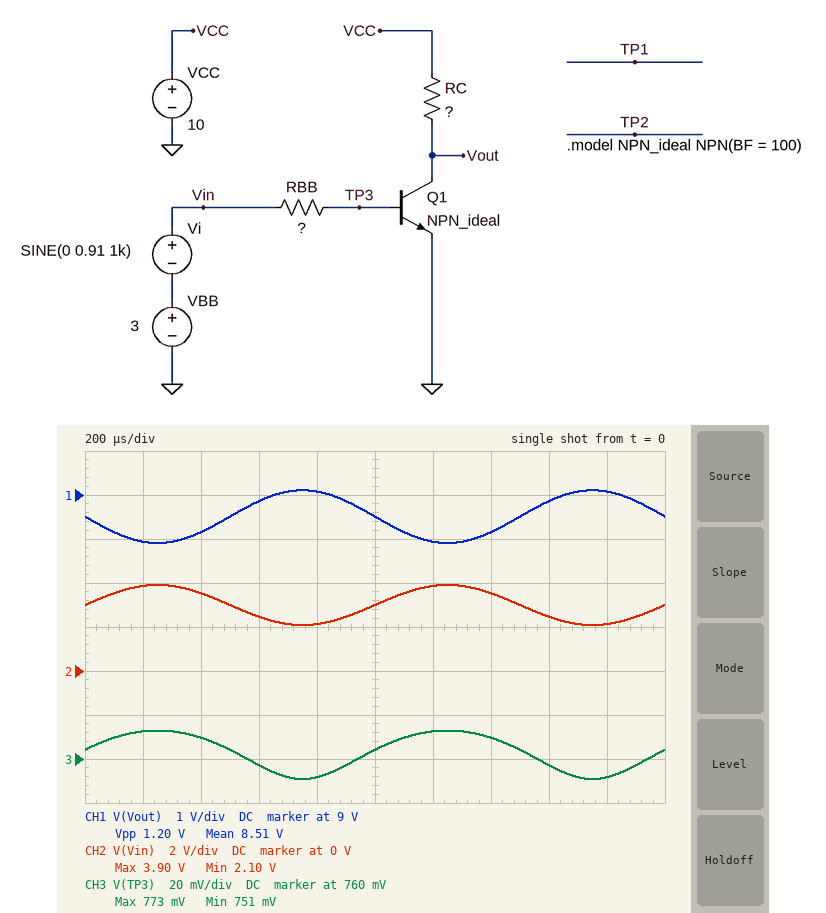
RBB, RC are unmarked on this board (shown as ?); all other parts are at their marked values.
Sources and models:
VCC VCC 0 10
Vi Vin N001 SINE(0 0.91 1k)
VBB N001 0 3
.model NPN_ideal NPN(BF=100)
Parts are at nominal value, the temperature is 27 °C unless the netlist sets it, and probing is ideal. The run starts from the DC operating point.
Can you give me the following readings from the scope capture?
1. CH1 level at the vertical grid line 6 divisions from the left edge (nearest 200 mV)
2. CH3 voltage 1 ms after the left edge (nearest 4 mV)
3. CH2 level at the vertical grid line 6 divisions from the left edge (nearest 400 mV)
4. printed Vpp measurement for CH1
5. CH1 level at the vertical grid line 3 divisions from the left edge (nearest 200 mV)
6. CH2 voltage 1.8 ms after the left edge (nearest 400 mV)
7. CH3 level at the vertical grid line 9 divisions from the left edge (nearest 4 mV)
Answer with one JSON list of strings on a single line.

["8.0 V", "764 mV", "4.0 V", "1.20 V", "8.8 V", "2.0 V", "752 mV"]
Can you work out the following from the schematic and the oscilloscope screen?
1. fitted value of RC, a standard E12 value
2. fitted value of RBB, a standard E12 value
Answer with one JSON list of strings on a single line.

["2.2 kΩ", "330 kΩ"]
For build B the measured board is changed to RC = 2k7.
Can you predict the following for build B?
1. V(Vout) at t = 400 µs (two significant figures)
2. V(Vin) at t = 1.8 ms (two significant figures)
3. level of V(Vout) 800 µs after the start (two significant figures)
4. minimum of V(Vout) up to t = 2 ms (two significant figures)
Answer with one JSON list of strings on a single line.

["7.7 V", "2.1 V", "8.9 V", "7.4 V"]
